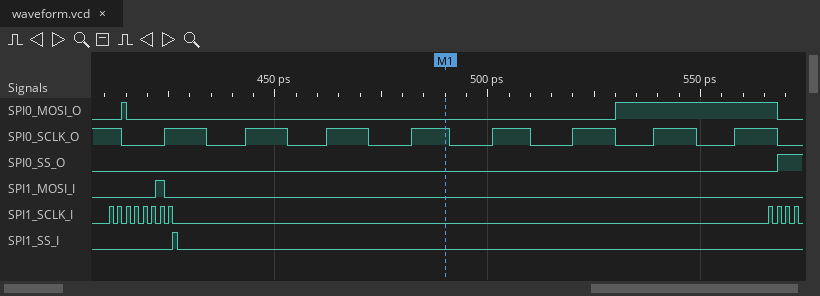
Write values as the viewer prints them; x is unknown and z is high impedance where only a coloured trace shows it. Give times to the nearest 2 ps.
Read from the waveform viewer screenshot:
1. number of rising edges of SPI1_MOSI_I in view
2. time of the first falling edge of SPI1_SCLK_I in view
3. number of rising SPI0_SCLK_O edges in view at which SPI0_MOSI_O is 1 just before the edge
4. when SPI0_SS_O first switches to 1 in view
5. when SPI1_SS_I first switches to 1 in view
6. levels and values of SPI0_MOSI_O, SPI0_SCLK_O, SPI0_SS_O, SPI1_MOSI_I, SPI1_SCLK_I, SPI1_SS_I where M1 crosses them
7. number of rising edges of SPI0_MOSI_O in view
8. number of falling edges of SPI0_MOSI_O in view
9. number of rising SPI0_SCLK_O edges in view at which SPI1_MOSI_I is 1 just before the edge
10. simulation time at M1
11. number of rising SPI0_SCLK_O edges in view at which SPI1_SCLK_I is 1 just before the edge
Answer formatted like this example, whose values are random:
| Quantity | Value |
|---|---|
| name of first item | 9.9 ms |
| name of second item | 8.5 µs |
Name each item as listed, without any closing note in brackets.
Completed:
| Quantity | Value |
|---|---|
| number of rising edges of SPI1_MOSI_I in view | 1 |
| time of the first falling edge of SPI1_SCLK_I in view | 412 ps |
| number of rising SPI0_SCLK_O edges in view at which SPI0_MOSI_O is 1 just before the edge | 2 |
| when SPI0_SS_O first switches to 1 in view | 568 ps |
| when SPI1_SS_I first switches to 1 in view | 426 ps |
| levels and values of SPI0_MOSI_O, SPI0_SCLK_O, SPI0_SS_O, SPI1_MOSI_I, SPI1_SCLK_I, SPI1_SS_I where M1 crosses them | SPI0_MOSI_O=0, SPI0_SCLK_O=1, SPI0_SS_O=0, SPI1_MOSI_I=0, SPI1_SCLK_I=0, SPI1_SS_I=0 |
| number of rising edges of SPI0_MOSI_O in view | 2 |
| number of falling edges of SPI0_MOSI_O in view | 2 |
| number of rising SPI0_SCLK_O edges in view at which SPI1_MOSI_I is 1 just before the edge | 1 |
| simulation time at M1 | 490 ps |
| number of rising SPI0_SCLK_O edges in view at which SPI1_SCLK_I is 1 just before the edge | 1 |
